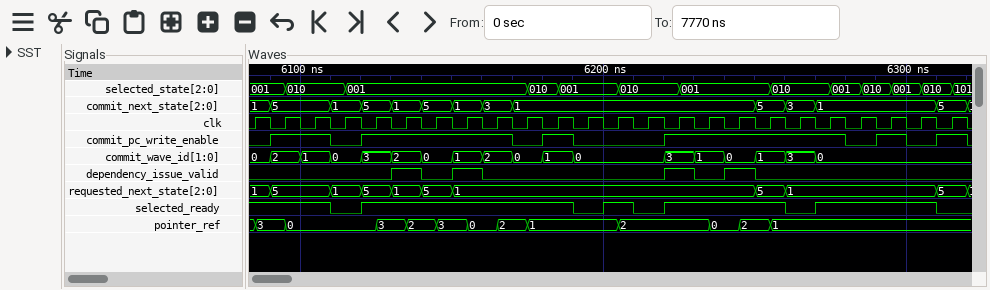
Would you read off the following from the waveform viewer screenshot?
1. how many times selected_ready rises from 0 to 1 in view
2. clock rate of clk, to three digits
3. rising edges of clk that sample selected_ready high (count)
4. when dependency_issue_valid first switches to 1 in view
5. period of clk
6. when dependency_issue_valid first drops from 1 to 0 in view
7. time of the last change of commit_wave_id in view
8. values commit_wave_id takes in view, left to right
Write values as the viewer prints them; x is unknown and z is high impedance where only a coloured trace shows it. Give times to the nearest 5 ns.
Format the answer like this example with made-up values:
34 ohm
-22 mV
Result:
4
100 MHz
19
6130 ns
10 ns
6140 ns
6270 ns
0, 2, 1, 0, 3, 2, 0, 1, 2, 0, 1, 0, 3, 1, 0, 1, 3, 0
